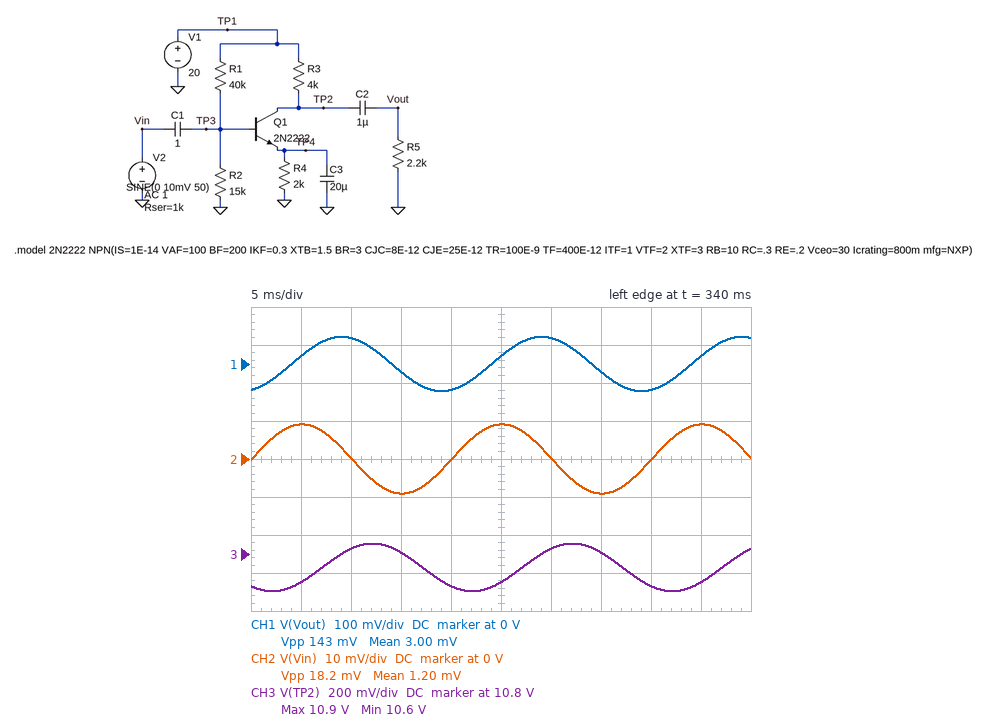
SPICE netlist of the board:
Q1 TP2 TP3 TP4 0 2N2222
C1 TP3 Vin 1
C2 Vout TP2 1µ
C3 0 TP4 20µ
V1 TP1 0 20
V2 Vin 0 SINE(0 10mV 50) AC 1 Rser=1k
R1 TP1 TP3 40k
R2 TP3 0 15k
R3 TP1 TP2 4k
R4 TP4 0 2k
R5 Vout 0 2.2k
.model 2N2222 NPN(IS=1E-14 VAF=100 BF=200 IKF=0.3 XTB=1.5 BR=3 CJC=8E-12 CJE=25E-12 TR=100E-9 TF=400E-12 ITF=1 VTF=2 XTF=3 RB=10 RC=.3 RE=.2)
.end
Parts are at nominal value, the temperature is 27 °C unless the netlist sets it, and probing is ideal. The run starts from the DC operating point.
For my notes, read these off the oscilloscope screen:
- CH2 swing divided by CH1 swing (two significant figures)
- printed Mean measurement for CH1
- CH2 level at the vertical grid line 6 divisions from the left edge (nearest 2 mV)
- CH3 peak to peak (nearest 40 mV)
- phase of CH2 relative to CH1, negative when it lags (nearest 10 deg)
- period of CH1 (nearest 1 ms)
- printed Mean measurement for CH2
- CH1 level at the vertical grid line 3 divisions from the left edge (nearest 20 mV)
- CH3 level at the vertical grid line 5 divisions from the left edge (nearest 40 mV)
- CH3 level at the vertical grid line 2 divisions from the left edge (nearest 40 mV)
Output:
0.13
3.00 mV
0 V
240 mV
70 deg
20 ms
1.20 mV
-20 mV
10.64 V
10.84 V
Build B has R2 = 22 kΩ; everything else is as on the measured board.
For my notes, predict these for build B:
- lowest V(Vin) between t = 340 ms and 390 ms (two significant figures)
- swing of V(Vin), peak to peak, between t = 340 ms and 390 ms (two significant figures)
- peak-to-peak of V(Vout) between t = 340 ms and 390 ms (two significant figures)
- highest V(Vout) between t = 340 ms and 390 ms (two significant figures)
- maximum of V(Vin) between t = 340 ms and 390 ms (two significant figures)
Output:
-9.3 mV
19 mV
150 mV
73 mV
9.3 mV
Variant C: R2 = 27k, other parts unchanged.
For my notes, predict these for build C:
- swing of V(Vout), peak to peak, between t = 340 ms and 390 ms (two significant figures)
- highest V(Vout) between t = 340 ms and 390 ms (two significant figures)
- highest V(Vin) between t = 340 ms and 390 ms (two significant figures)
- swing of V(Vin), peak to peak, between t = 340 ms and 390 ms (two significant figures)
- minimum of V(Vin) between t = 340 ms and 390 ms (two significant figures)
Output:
9.9 mV
4.9 mV
1.9 mV
4.1 mV
-2.1 mV
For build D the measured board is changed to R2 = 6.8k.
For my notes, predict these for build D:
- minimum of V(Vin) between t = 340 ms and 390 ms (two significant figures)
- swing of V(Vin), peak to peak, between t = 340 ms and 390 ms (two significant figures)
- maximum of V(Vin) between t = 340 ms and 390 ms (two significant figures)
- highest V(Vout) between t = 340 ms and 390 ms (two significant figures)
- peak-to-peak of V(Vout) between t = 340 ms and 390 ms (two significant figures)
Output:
-8.5 mV
17 mV
8.5 mV
65 mV
130 mV
